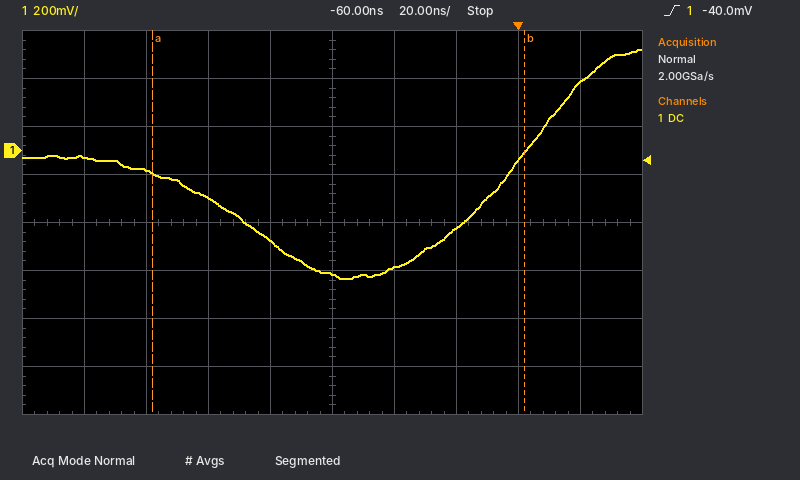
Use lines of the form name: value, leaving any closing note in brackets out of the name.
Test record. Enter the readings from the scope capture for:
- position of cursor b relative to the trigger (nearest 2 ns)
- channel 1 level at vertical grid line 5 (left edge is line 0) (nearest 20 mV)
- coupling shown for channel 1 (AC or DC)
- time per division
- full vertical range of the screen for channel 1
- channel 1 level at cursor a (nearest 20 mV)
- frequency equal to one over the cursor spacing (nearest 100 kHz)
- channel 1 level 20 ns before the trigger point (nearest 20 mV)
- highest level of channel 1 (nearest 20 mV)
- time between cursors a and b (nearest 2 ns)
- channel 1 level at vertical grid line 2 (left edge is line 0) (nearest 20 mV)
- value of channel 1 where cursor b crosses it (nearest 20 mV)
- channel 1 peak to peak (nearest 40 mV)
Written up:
position of cursor b relative to the trigger: +2 ns
channel 1 level at vertical grid line 5 (left edge is line 0): -520 mV
coupling shown for channel 1: DC
time per division: 20 ns
full vertical range of the screen for channel 1: 1.6 V
channel 1 level at cursor a: -100 mV
frequency equal to one over the cursor spacing: 8.3 MHz
channel 1 level 20 ns before the trigger point: -320 mV
highest level of channel 1: 420 mV
time between cursors a and b: 120 ns
channel 1 level at vertical grid line 2 (left edge is line 0): -80 mV
value of channel 1 where cursor b crosses it: 0 mV
channel 1 peak to peak: 960 mV
